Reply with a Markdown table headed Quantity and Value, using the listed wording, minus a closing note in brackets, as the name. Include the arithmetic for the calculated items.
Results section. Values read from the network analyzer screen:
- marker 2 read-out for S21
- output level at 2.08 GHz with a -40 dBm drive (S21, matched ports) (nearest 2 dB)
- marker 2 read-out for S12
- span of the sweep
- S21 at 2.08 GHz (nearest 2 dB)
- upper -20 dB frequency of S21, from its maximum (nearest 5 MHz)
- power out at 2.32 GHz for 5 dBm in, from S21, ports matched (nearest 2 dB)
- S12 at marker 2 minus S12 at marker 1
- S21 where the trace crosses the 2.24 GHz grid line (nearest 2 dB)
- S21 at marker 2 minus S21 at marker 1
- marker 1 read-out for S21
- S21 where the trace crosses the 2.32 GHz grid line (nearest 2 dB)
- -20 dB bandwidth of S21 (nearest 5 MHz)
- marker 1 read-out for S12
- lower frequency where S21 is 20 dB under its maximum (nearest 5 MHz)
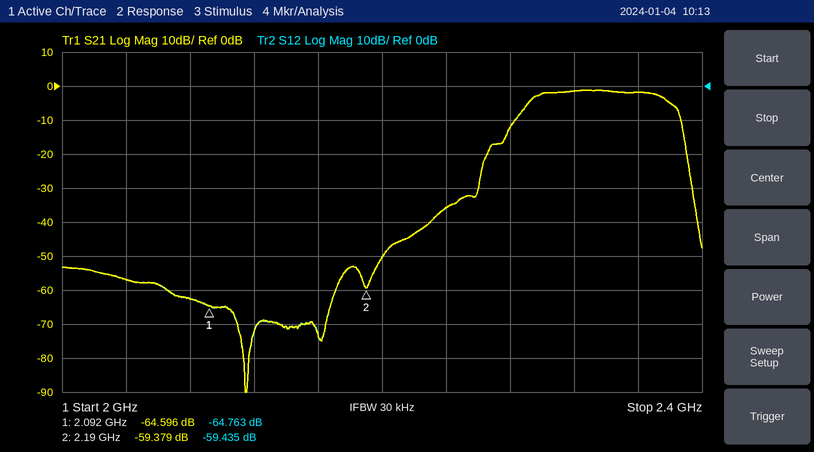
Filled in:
| Quantity | Value |
|---|---|
| marker 2 read-out for S21 | -59.379 dB |
| output level at 2.08 GHz with a -40 dBm drive (S21, matched ports) | -40 dBm + (-62 dB) = -102 dBm |
| marker 2 read-out for S12 | -59.435 dB |
| span of the sweep | 400 MHz |
| S21 at 2.08 GHz | -62 dB |
| upper -20 dB frequency of S21, from its maximum | 2.390 GHz |
| power out at 2.32 GHz for 5 dBm in, from S21, ports matched | 5 dBm + (-2 dB) = 4 dBm |
| S12 at marker 2 minus S12 at marker 1 | -59.435 − (-64.763) = 5.328 dB |
| S21 where the trace crosses the 2.24 GHz grid line | -36 dB |
| S21 at marker 2 minus S21 at marker 1 | -59.379 − (-64.596) = 5.217 dB |
| marker 1 read-out for S21 | -64.596 dB |
| S21 where the trace crosses the 2.32 GHz grid line | -2 dB |
| -20 dB bandwidth of S21 | 2.390 GHz − 2.265 GHz = 125 MHz |
| marker 1 read-out for S12 | -64.763 dB |
| lower frequency where S21 is 20 dB under its maximum | 2.265 GHz |
